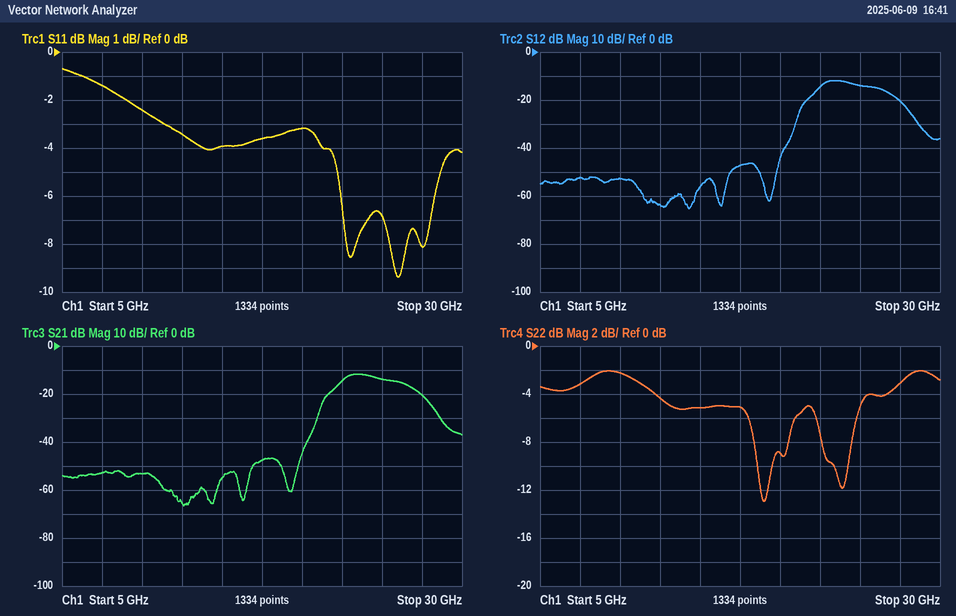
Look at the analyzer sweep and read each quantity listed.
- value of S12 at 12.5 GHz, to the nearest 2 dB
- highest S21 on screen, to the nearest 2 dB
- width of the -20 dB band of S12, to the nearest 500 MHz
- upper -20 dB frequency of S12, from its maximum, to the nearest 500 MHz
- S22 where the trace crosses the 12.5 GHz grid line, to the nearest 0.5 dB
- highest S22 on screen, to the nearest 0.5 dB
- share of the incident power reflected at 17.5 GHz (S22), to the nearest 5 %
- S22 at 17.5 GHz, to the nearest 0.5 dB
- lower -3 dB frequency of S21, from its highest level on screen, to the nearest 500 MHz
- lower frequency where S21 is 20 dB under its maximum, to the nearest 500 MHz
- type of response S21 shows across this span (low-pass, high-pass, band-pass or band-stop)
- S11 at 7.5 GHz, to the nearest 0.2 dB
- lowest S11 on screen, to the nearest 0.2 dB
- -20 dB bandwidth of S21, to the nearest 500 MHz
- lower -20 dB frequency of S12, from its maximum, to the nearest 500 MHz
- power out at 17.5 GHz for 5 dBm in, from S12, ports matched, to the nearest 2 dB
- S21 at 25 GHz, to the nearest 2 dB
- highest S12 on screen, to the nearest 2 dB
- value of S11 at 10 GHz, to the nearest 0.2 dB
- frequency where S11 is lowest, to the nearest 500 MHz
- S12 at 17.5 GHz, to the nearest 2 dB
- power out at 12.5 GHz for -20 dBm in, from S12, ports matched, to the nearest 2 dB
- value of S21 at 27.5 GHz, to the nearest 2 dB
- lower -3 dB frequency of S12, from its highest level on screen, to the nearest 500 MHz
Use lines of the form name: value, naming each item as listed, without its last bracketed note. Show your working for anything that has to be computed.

value of S12 at 12.5 GHz, to the nearest 2 dB: -64 dB
highest S21 on screen, to the nearest 2 dB: -12 dB
width of the -20 dB band of S12, to the nearest 500 MHz: 29.0 GHz − 21.0 GHz = 8.0 GHz
upper -20 dB frequency of S12, from its maximum, to the nearest 500 MHz: 29.0 GHz
S22 where the trace crosses the 12.5 GHz grid line, to the nearest 0.5 dB: -4.5 dB
highest S22 on screen, to the nearest 0.5 dB: -2.0 dB
share of the incident power reflected at 17.5 GHz (S22), to the nearest 5 %: 10^(-5/10) ≈ 31.6 %, so 30 % to the nearest 5 %
S22 at 17.5 GHz, to the nearest 0.5 dB: -5.0 dB
lower -3 dB frequency of S21, from its highest level on screen, to the nearest 500 MHz: 22.5 GHz
lower frequency where S21 is 20 dB under its maximum, to the nearest 500 MHz: 21.0 GHz
type of response S21 shows across this span: band-pass
S11 at 7.5 GHz, to the nearest 0.2 dB: -1.4 dB
lowest S11 on screen, to the nearest 0.2 dB: -9.4 dB
-20 dB bandwidth of S21, to the nearest 500 MHz: 29.0 GHz − 21.0 GHz = 8.0 GHz
lower -20 dB frequency of S12, from its maximum, to the nearest 500 MHz: 21.0 GHz
power out at 17.5 GHz for 5 dBm in, from S12, ports matched, to the nearest 2 dB: 5 dBm + (-48 dB) = -42 dBm
S21 at 25 GHz, to the nearest 2 dB: -14 dB
highest S12 on screen, to the nearest 2 dB: -12 dB
value of S11 at 10 GHz, to the nearest 0.2 dB: -2.4 dB
frequency where S11 is lowest, to the nearest 500 MHz: 26.0 GHz
S12 at 17.5 GHz, to the nearest 2 dB: -48 dB
power out at 12.5 GHz for -20 dBm in, from S12, ports matched, to the nearest 2 dB: -20 dBm + (-64 dB) = -84 dBm
value of S21 at 27.5 GHz, to the nearest 2 dB: -20 dB
lower -3 dB frequency of S12, from its highest level on screen, to the nearest 500 MHz: 22.5 GHz
